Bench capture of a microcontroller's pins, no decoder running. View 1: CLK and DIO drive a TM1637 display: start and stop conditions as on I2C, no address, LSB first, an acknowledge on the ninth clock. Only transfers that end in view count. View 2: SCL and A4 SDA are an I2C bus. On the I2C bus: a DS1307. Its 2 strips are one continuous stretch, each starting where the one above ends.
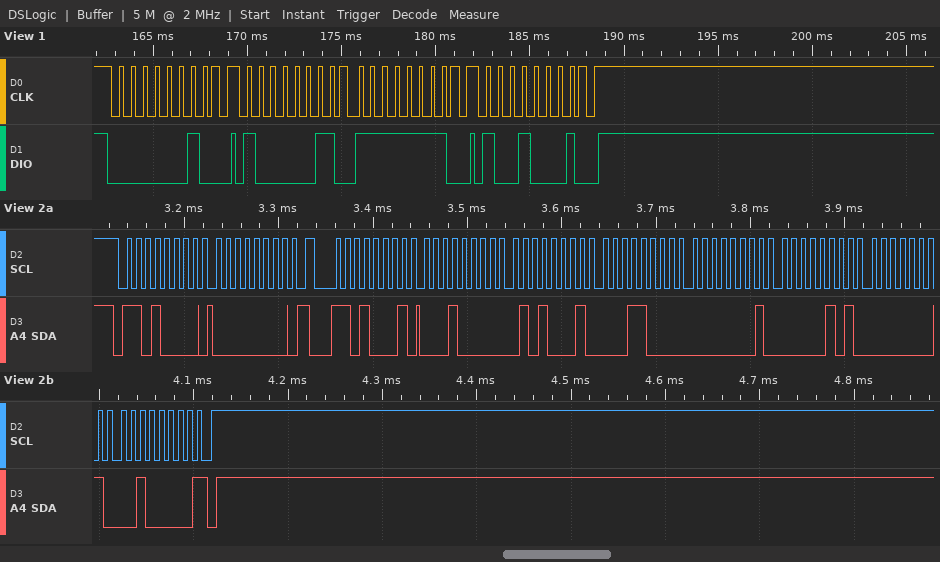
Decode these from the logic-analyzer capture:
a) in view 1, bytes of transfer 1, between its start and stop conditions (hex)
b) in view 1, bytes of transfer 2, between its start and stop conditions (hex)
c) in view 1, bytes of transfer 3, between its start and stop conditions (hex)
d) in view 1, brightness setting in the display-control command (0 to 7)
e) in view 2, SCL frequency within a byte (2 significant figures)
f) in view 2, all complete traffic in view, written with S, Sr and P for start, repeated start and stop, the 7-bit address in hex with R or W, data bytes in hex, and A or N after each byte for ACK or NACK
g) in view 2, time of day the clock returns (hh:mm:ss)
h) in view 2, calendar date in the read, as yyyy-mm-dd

40
C1 FF
89
1
100 kHz
S 68W A 00 A Sr 68R A 10 A 51 A 18 A 01 A 05 A 01 A 20 N P
18:51:10
2020-01-05
